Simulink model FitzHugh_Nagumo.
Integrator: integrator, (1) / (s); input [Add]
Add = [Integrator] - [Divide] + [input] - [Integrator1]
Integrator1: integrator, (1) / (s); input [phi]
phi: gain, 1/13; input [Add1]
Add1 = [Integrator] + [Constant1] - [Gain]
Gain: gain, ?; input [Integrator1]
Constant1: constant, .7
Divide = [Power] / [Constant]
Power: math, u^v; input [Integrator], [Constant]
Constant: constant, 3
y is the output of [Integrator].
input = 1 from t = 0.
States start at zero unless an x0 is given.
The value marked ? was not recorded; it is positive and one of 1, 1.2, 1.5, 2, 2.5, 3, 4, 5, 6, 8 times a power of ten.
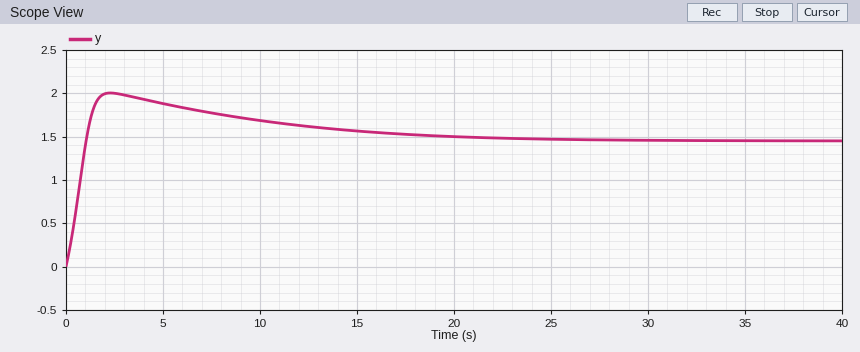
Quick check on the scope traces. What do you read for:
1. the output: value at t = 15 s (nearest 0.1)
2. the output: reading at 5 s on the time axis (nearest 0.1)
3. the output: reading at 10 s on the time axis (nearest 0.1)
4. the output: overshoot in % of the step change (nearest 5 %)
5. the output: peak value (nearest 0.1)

1.6
1.9
1.7
40 %
2.0
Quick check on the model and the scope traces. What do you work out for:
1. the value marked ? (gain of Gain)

1.5
